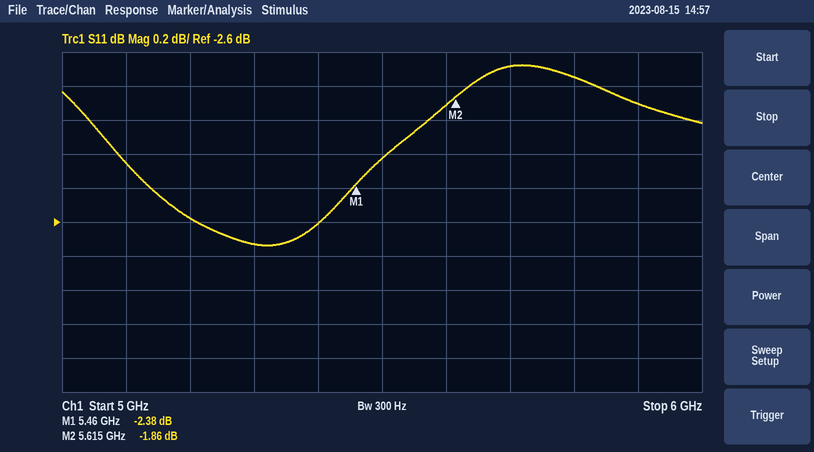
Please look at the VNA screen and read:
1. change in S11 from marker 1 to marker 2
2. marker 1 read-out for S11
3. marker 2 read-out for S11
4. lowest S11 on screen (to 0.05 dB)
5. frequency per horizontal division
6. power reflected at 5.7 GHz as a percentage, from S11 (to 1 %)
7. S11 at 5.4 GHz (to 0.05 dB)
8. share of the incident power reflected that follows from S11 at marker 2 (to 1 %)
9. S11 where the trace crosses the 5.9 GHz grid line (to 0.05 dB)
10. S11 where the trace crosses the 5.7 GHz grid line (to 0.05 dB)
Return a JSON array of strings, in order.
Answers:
["0.52 dB", "-2.38 dB", "-1.86 dB", "-2.75 dB", "100 MHz", "68 %", "-2.60 dB", "65 %", "-1.90 dB", "-1.70 dB"]
